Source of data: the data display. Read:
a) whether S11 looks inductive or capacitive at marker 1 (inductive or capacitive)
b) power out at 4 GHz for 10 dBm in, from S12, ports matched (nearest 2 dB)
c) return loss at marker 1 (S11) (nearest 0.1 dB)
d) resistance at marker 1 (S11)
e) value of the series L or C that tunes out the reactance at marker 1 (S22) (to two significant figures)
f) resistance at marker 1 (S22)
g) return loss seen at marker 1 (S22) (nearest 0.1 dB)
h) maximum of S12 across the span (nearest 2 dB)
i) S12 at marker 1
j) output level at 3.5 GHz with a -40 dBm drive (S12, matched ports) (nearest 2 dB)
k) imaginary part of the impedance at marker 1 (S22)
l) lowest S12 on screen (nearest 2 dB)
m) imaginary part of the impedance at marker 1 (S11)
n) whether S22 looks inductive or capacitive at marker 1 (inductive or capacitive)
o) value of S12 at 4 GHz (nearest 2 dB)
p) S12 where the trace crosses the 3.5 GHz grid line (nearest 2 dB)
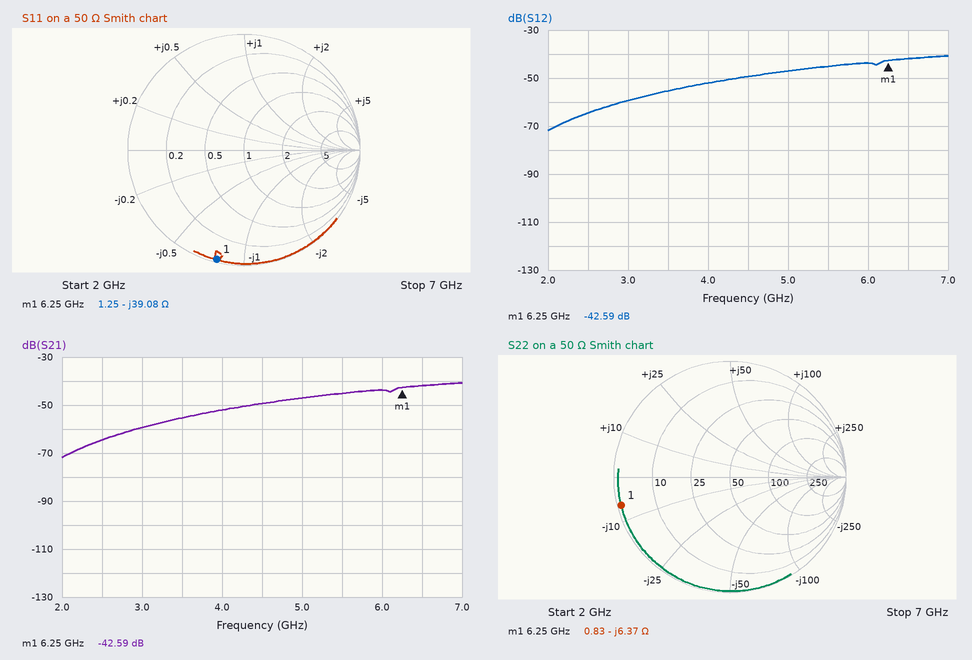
capacitive
-42 dBm
0.3 dB
1.25 Ω
160 pH
0.83 Ω
0.3 dB
-40 dB
-42.59 dB
-96 dBm
-6.37 Ω
-72 dB
-39.08 Ω
capacitive
-52 dB
-56 dB
